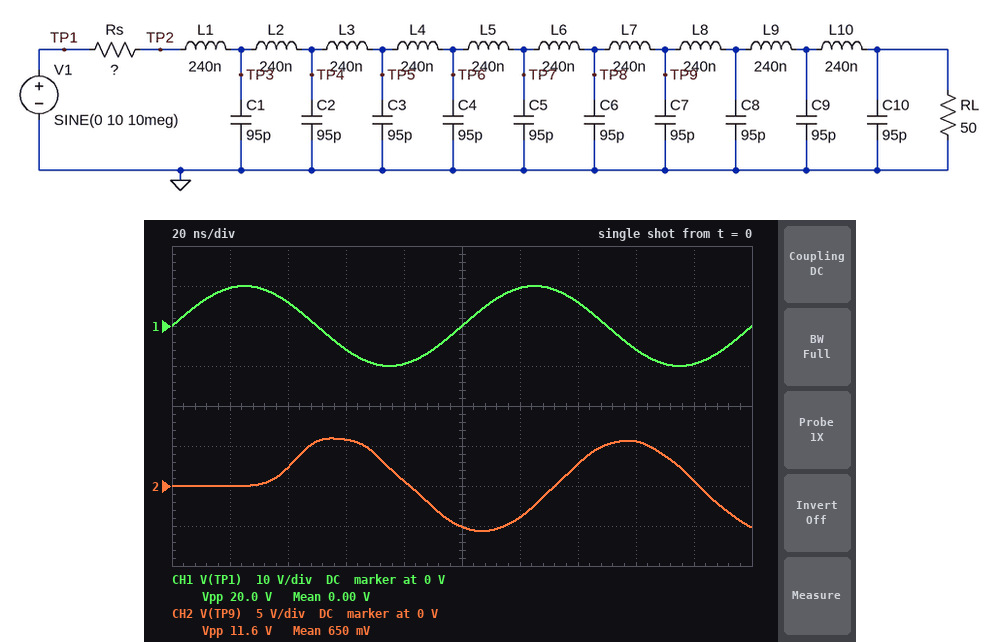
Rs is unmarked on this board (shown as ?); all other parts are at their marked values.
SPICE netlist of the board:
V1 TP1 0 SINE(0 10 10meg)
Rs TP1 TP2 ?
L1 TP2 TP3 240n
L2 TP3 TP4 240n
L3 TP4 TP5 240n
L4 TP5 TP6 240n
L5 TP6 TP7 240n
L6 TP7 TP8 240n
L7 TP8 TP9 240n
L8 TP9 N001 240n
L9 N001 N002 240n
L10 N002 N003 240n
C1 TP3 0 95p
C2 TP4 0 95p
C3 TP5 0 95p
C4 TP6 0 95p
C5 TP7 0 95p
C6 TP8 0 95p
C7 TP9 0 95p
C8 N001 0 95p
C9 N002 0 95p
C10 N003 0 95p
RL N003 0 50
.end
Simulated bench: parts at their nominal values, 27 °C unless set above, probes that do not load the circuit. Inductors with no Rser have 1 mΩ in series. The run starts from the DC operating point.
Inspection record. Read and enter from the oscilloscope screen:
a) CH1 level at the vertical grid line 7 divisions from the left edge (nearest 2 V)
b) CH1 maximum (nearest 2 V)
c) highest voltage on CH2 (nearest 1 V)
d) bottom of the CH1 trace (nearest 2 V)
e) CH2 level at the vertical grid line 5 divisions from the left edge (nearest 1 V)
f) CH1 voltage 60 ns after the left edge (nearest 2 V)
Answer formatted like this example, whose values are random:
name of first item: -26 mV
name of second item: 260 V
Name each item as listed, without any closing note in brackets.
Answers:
CH1 level at the vertical grid line 7 divisions from the left edge: 6 V
CH1 maximum: 10 V
highest voltage on CH2: 6 V
bottom of the CH1 trace: -10 V
CH2 level at the vertical grid line 5 divisions from the left edge: -5 V
CH1 voltage 60 ns after the left edge: -6 V
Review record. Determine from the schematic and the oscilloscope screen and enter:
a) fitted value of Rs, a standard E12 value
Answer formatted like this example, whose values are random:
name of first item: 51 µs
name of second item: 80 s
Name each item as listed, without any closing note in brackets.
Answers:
fitted value of Rs, a standard E12 value: 33 Ω
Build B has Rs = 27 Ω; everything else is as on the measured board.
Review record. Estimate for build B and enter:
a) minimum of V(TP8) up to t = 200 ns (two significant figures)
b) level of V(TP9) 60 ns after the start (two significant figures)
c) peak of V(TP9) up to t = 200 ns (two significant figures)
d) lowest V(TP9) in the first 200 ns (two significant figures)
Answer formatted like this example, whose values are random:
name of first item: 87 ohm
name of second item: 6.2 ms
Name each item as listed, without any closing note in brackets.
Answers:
minimum of V(TP8) up to t = 200 ns: -6.4 V
level of V(TP9) 60 ns after the start: 6.2 V
peak of V(TP9) up to t = 200 ns: 6.4 V
lowest V(TP9) in the first 200 ns: -6.1 V
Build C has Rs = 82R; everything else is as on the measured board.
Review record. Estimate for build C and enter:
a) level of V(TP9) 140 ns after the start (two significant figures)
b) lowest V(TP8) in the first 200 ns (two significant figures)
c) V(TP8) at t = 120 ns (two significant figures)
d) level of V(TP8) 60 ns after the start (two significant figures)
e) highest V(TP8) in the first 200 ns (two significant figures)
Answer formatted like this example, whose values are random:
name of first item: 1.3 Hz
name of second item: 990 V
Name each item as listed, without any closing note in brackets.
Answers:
level of V(TP9) 140 ns after the start: 1.7 V
lowest V(TP8) in the first 200 ns: -3.7 V
V(TP8) at t = 120 ns: -1.4 V
level of V(TP8) 60 ns after the start: 3.4 V
highest V(TP8) in the first 200 ns: 3.7 V
